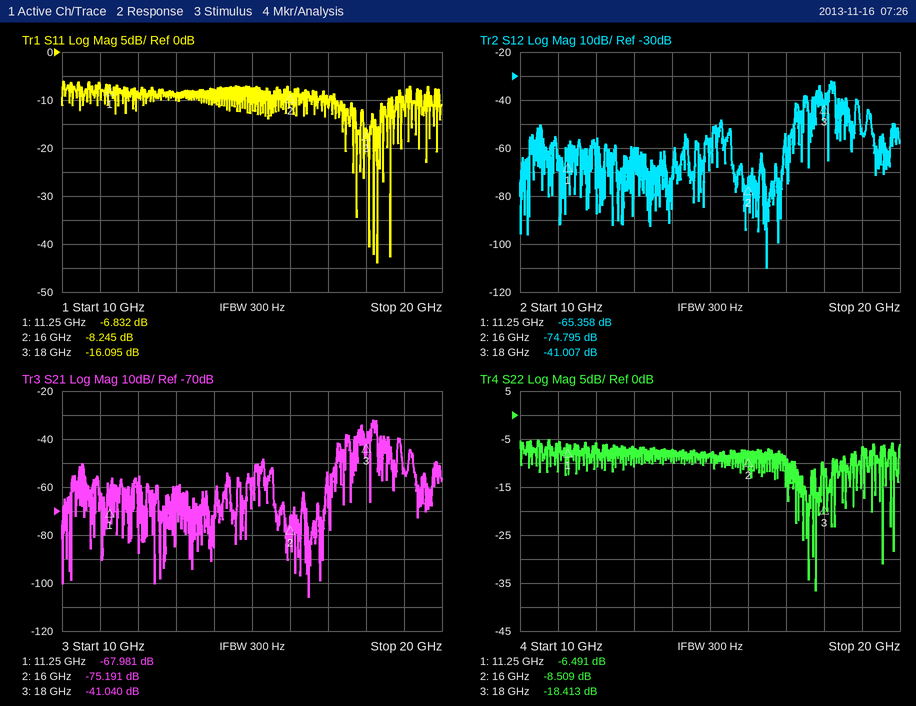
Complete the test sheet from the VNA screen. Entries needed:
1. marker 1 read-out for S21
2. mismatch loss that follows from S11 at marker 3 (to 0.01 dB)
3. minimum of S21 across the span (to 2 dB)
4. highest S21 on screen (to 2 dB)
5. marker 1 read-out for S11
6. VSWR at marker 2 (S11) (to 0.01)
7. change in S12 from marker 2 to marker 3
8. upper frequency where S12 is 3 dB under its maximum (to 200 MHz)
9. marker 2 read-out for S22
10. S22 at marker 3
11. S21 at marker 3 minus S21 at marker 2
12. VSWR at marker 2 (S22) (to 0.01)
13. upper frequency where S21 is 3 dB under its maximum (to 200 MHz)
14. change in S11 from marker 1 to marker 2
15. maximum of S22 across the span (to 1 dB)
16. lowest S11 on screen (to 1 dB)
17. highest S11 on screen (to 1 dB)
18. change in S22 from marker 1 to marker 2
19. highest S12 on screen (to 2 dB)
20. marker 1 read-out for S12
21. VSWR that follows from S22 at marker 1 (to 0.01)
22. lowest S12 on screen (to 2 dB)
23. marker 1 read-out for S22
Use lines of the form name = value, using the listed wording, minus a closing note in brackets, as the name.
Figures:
marker 1 read-out for S21 = -67.981 dB
mismatch loss that follows from S11 at marker 3 = 0.11 dB
minimum of S21 across the span = -106 dB
highest S21 on screen = -32 dB
marker 1 read-out for S11 = -6.832 dB
VSWR at marker 2 (S11) = 2.26
change in S12 from marker 2 to marker 3 = 33.788 dB
upper frequency where S12 is 3 dB under its maximum = 18.2 GHz
marker 2 read-out for S22 = -8.509 dB
S22 at marker 3 = -18.413 dB
S21 at marker 3 minus S21 at marker 2 = 34.151 dB
VSWR at marker 2 (S22) = 2.20
upper frequency where S21 is 3 dB under its maximum = 18.2 GHz
change in S11 from marker 1 to marker 2 = -1.413 dB
maximum of S22 across the span = -5 dB
lowest S11 on screen = -44 dB
highest S11 on screen = -6 dB
change in S22 from marker 1 to marker 2 = -2.018 dB
highest S12 on screen = -32 dB
marker 1 read-out for S12 = -65.358 dB
VSWR that follows from S22 at marker 1 = 2.80
lowest S12 on screen = -110 dB
marker 1 read-out for S22 = -6.491 dB
